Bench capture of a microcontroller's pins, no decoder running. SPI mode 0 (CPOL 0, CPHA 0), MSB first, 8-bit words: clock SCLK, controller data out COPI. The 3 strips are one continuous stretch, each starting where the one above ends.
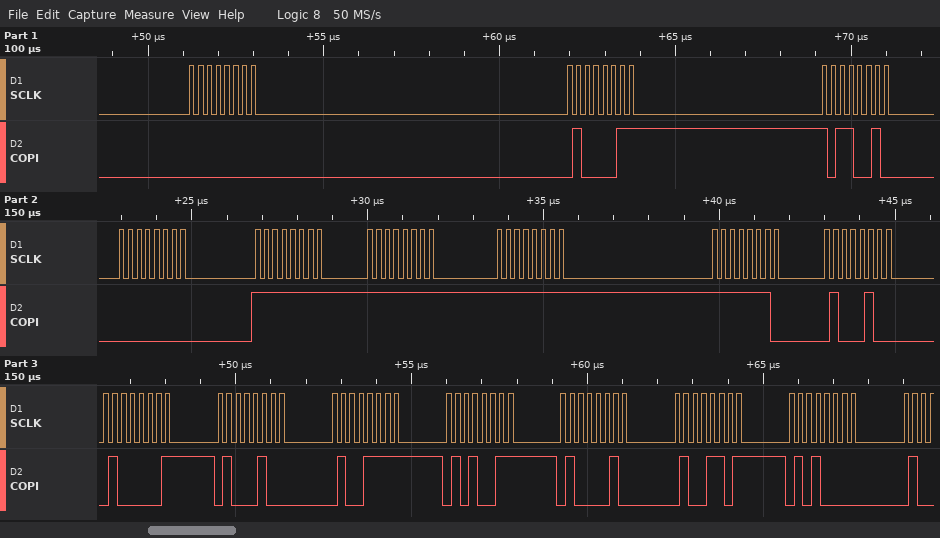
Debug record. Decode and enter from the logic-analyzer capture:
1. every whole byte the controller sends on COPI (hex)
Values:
00 43 B2 00 FF FF FF FE 44 41 44 4F 53 42 4D 50
